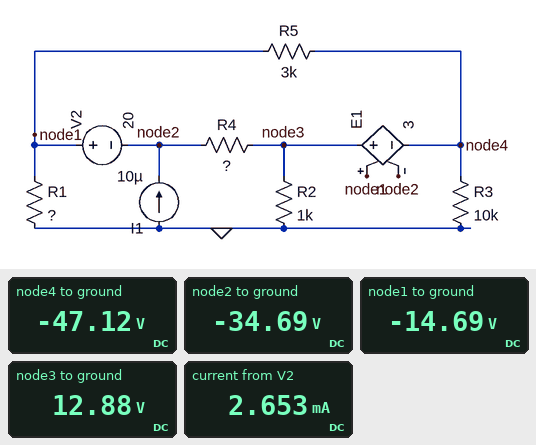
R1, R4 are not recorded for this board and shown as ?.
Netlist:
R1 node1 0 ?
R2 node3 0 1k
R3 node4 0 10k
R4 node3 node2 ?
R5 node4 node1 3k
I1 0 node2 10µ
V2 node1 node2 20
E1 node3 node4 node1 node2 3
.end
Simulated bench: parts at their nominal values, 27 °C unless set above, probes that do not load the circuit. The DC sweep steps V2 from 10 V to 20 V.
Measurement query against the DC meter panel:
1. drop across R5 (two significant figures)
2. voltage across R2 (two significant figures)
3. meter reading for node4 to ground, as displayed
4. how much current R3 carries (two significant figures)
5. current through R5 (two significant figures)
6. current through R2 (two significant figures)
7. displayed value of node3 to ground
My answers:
32 V
13 V
-47.12 V
4.7 mA
11 mA
13 mA
12.88 V
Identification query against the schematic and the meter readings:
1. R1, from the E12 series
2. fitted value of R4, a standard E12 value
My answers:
1.8 kΩ
18 kΩ
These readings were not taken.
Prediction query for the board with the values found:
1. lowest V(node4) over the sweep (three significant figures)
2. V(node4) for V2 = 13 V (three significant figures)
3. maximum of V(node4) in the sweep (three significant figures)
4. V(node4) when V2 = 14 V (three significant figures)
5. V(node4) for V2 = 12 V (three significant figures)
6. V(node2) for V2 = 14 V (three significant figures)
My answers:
-47.1 V
-30.6 V
-23.6 V
-33.0 V
-28.3 V
-24.3 V
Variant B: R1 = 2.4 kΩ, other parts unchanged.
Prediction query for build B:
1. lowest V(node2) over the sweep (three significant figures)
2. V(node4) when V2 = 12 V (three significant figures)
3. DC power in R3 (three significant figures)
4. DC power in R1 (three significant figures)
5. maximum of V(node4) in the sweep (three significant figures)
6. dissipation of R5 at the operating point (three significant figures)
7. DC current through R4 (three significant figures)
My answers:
-37.6 V
-28.7 V
229 mW
129 mW
-23.9 V
306 mW
2.76 mA
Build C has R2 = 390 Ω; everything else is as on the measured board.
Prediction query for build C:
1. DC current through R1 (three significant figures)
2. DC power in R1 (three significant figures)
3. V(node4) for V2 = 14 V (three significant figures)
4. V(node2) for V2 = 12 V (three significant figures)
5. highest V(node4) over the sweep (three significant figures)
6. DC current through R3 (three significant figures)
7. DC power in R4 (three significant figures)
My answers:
9.75 mA
171 mW
-37.9 V
-22.5 V
-27.0 V
5.41 mA
105 mW
